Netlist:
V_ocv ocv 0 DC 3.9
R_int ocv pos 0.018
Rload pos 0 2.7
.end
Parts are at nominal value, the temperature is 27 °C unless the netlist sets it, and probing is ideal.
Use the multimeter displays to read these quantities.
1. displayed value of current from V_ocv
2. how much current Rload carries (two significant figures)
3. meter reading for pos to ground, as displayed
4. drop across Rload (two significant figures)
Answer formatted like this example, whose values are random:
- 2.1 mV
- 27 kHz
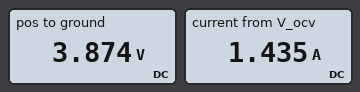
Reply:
- 1.435 A
- 1.4 A
- 3.874 V
- 3.9 V
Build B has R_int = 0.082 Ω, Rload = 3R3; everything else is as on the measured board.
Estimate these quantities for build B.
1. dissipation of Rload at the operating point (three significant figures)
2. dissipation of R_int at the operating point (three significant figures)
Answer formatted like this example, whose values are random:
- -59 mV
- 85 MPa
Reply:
- 4.39 W
- 109 mW
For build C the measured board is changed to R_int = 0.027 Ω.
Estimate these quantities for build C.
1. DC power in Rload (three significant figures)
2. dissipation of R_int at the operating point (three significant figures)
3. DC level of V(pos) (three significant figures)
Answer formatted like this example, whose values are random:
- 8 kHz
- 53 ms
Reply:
- 5.52 W
- 55.2 mW
- 3.86 V
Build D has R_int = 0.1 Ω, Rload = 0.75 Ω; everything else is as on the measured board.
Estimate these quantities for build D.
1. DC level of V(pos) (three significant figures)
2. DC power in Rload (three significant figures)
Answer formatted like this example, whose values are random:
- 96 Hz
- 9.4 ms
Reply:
- 3.44 V
- 15.8 W
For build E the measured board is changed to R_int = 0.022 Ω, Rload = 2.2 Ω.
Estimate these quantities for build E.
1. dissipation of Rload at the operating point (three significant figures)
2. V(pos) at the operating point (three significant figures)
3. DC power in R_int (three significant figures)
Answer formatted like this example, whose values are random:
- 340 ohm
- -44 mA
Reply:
- 6.78 W
- 3.86 V
- 67.8 mW
